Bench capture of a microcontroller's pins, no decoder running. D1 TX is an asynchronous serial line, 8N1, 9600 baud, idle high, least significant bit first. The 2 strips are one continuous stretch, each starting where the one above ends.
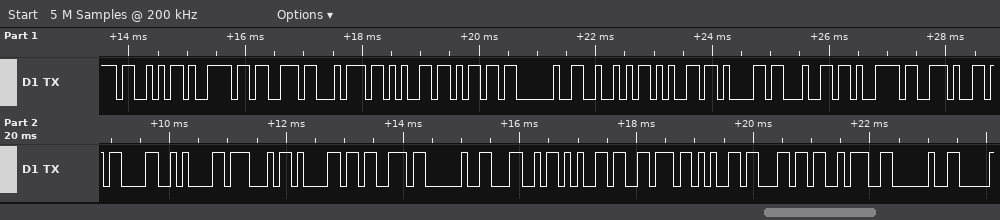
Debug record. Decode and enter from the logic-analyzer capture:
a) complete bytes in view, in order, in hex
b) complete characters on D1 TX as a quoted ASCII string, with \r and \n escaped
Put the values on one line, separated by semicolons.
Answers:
0x53 0x79 0x73 0x74 0x65 0x6D 0x20 0x52 0x65 0x61 0x64 0x79 0x2E 0x0D 0x0A 0x47 0x61 0x73 0x20 0x4C 0x65 0x76 0x65 0x6C 0x3A 0x20; "System Ready.\r\nGas Level: "
